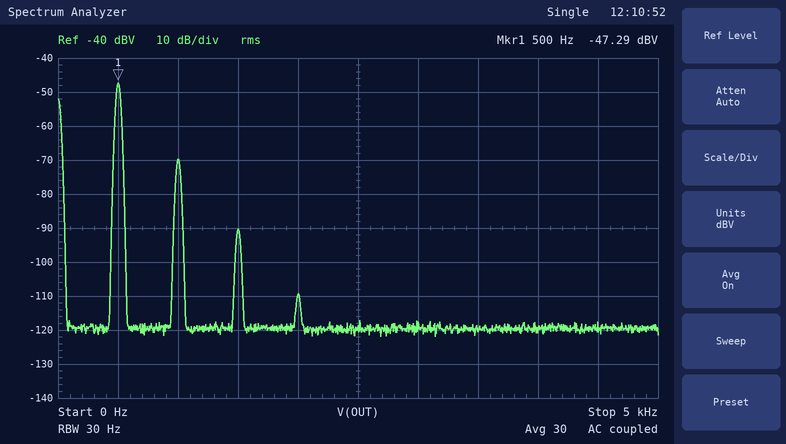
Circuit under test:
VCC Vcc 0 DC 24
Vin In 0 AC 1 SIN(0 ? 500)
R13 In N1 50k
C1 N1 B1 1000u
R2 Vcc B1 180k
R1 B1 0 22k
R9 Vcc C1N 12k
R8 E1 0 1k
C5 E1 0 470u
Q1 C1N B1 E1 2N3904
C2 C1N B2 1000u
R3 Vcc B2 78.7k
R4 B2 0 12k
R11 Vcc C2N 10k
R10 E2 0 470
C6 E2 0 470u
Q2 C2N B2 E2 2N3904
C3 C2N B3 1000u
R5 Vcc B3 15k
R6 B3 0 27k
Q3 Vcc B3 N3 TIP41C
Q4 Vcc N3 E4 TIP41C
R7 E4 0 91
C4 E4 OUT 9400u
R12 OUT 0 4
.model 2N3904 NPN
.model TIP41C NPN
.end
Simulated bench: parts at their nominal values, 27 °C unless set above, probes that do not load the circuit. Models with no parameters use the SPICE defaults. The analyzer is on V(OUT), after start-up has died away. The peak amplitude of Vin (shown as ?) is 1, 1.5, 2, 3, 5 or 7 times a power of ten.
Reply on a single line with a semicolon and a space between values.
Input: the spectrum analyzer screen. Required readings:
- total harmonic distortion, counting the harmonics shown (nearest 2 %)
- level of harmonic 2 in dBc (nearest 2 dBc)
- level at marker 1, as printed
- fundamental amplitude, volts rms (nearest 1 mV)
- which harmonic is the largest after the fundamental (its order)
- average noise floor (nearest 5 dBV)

8 %; -22 dBc; -47.29 dBV; 4 mV; 2; -120 dBV
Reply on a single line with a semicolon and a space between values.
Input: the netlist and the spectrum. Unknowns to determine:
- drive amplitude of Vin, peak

15 mV
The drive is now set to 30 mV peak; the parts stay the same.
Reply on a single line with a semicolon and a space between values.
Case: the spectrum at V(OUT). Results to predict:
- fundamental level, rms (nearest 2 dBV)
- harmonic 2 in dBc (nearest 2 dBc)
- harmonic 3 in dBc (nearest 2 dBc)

-40 dBV; -16 dBc; -30 dBc
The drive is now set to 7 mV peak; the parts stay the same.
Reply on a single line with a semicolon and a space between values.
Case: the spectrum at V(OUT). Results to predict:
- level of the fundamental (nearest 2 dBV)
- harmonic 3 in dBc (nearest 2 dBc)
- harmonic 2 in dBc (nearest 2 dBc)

-54 dBV; -56 dBc; -30 dBc
